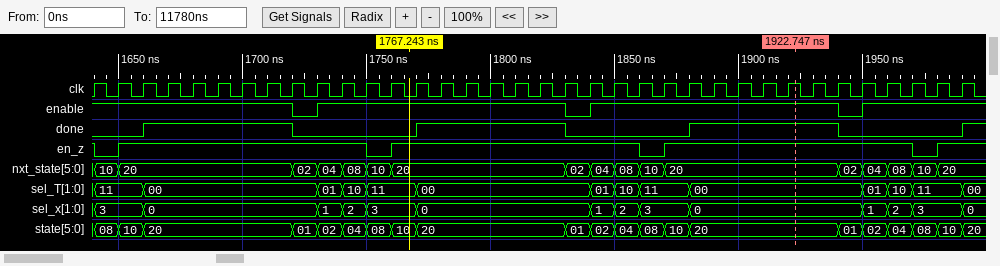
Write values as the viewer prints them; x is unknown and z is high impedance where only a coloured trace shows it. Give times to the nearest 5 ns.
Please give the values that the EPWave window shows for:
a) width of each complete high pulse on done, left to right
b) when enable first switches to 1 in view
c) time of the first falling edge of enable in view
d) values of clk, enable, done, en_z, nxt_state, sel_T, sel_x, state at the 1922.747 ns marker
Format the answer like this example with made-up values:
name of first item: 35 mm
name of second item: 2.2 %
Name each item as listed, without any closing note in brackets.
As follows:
width of each complete high pulse on done, left to right: 60 ns, 60 ns, 60 ns
when enable first switches to 1 in view: 1730 ns
time of the first falling edge of enable in view: 1720 ns
values of clk, enable, done, en_z, nxt_state, sel_T, sel_x, state at the 1922.747 ns marker: clk=1, enable=1, done=1, en_z=1, nxt_state=20, sel_T=00, sel_x=0, state=20
